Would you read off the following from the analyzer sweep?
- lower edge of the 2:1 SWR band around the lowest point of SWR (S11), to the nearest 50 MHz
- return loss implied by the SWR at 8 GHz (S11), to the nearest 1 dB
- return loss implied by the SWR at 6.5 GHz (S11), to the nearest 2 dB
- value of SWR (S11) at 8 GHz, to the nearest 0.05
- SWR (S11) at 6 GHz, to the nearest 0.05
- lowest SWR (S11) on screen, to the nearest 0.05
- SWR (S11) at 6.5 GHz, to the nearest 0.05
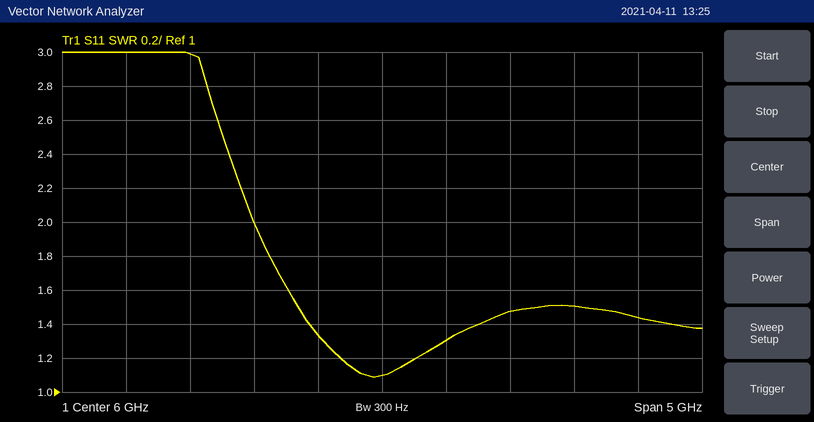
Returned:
5.00 GHz
15 dB
18 dB
1.45
1.10
1.10
1.30
